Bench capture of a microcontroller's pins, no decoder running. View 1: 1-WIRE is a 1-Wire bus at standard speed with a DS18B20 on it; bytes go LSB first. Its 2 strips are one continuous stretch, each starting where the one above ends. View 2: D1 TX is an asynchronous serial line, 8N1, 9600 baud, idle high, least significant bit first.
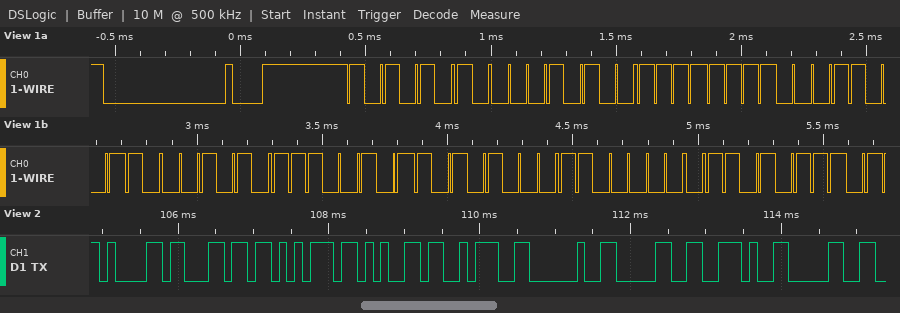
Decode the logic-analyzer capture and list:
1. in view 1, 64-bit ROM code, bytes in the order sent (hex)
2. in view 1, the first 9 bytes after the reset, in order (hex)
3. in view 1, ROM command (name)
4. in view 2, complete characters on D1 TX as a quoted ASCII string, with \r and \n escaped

28 FF 98 51 A7 15 03 EB
55 28 FF 98 51 A7 15 03 EB
Match ROM
"alue: 0.0"
